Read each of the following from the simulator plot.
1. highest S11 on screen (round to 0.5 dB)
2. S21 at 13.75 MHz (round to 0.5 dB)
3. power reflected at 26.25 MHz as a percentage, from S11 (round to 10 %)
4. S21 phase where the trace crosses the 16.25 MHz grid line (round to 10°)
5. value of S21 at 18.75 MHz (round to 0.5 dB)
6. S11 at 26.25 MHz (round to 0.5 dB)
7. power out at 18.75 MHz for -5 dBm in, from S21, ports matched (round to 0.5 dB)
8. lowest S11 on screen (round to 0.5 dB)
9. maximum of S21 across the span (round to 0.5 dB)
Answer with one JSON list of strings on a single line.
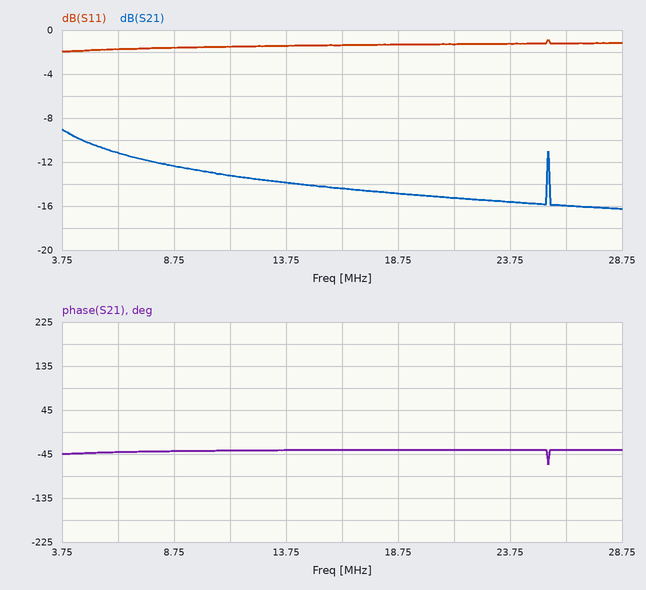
["-1.0 dB", "-14.0 dB", "80 %", "-40°", "-15.0 dB", "-1.0 dB", "-20.0 dBm", "-2.0 dB", "-9.0 dB"]
